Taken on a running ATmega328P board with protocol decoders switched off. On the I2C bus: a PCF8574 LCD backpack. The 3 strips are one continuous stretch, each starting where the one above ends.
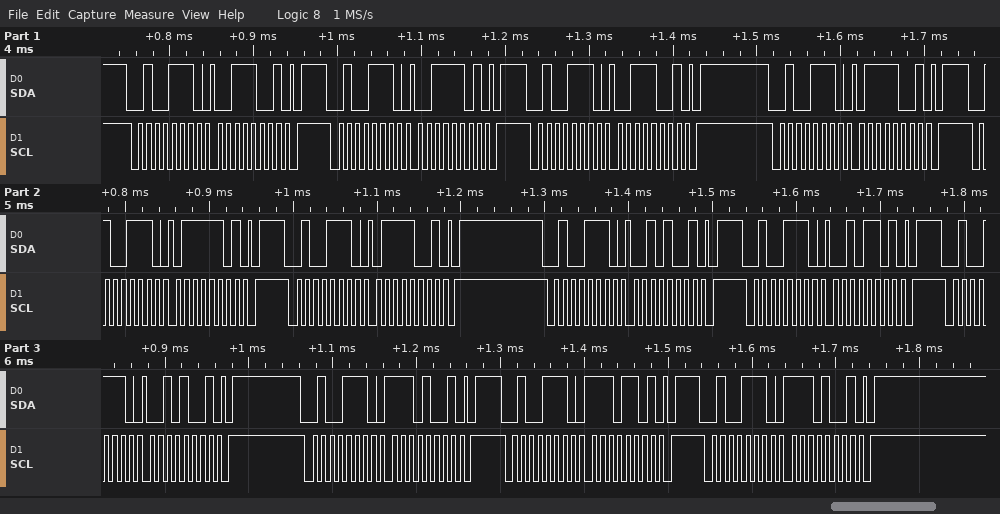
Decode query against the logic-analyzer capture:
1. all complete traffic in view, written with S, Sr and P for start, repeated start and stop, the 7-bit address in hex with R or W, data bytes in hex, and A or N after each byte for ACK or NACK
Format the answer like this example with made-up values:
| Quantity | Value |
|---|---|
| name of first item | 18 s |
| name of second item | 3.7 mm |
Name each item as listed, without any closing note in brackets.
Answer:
| Quantity | Value |
|---|---|
| all complete traffic in view, written with S, Sr and P for start, repeated start and stop, the 7-bit address in hex with R or W, data bytes in hex, and A or N after each byte for ACK or NACK | S 27W A 39 A P S 27W A 3D A P S 27W A 39 A P S 27W A 79 A P S 27W A 7D A P S 27W A 79 A P S 27W A 29 A P S 27W A 2D A P S 27W A 29 A P S 27W A E9 A P S 27W A ED A P S 27W A E9 A P |
